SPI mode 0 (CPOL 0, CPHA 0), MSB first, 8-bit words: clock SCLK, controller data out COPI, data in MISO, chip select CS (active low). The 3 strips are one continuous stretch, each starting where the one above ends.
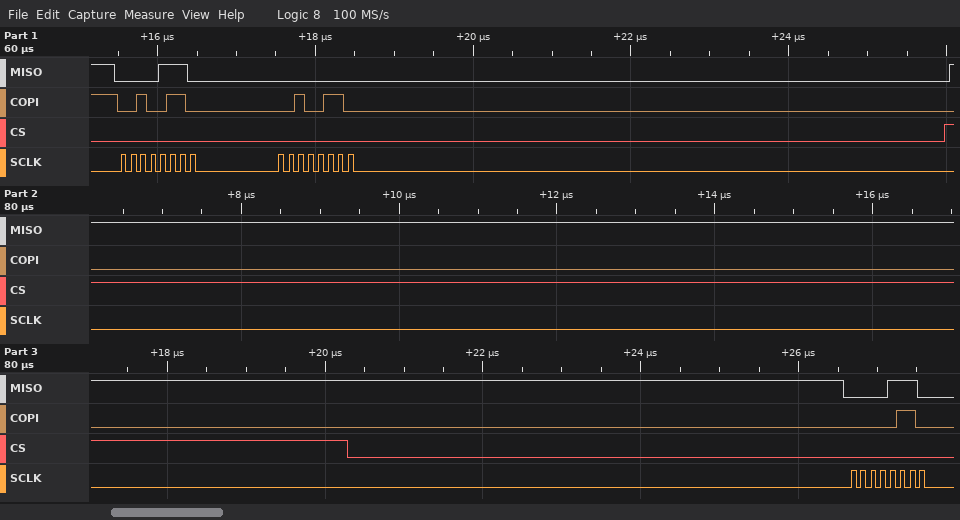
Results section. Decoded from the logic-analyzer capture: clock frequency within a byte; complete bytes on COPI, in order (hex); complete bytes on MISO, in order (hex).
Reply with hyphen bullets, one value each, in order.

- 8 MHz
- 26 26 06
- 0E 00 0E
